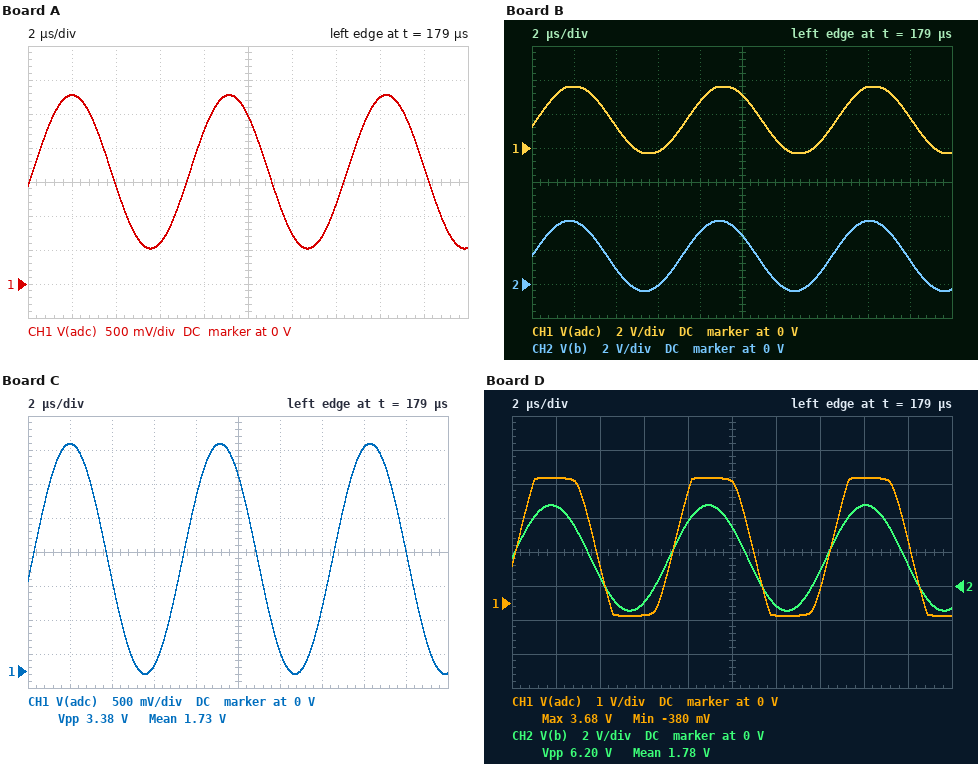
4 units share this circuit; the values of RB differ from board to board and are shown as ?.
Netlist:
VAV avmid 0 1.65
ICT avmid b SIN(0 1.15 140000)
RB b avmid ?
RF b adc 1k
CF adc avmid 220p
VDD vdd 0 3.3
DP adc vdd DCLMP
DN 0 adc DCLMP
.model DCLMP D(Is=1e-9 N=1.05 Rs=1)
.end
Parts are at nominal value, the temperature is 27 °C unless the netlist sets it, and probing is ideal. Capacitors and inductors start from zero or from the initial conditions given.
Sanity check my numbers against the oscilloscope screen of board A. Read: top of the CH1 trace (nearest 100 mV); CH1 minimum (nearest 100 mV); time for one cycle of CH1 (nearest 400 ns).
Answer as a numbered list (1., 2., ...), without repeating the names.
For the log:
1. 2.8 V
2. 500 mV
3. 7.2 µs
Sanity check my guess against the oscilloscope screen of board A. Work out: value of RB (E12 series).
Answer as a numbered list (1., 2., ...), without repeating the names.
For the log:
1. 1 Ω
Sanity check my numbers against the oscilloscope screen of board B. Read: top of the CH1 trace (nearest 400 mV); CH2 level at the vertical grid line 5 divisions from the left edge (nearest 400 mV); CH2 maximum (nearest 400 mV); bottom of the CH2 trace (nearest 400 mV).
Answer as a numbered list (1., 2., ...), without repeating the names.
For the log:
1. 3.6 V
2. 2.8 V
3. 3.6 V
4. -400 mV
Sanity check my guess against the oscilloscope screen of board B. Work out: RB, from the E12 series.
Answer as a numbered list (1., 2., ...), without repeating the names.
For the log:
1. 1.8 Ω
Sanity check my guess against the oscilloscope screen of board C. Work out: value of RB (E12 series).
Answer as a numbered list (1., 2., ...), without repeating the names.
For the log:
1. 1.5 Ω
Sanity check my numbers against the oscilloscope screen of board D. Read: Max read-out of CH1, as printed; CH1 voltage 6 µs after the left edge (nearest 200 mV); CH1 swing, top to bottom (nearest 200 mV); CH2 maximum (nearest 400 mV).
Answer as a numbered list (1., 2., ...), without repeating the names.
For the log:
1. 3.68 V
2. -400 mV
3. 4.0 V
4. 4.8 V
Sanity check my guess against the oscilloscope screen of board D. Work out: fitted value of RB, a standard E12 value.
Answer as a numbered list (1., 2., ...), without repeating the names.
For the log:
1. 2.7 Ω
